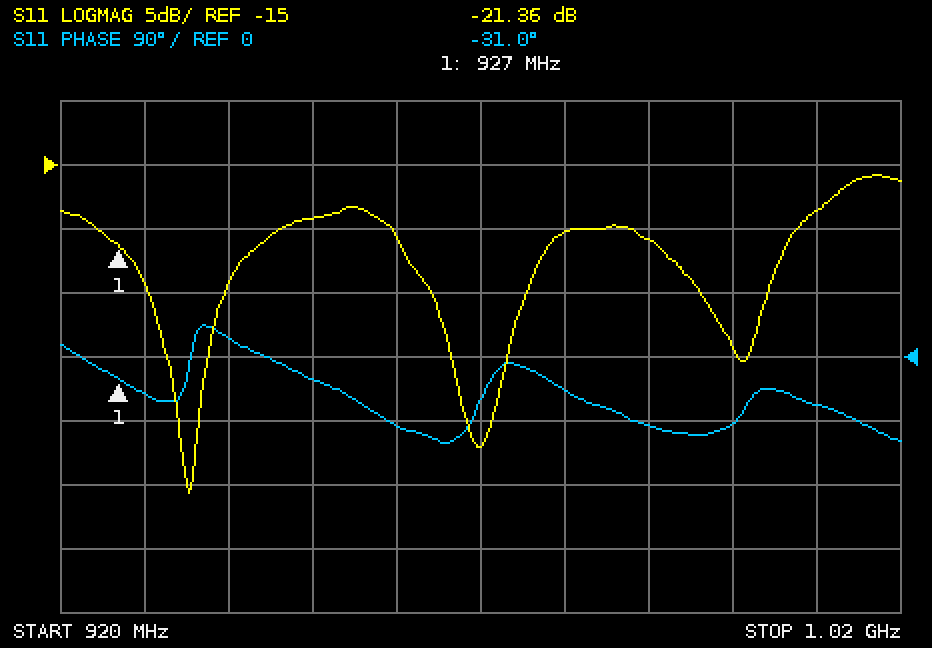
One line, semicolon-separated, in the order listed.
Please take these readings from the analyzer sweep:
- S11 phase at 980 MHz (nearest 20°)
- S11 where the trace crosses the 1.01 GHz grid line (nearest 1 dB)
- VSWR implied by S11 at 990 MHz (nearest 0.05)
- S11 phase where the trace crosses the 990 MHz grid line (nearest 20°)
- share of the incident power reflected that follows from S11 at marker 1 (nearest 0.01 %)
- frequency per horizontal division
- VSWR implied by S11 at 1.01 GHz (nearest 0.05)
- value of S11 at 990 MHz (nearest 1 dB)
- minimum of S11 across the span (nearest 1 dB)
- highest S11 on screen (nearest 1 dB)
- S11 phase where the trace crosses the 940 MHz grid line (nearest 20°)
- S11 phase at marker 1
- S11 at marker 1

-40°; -19 dB; 1.20; -100°; 0.73 %; 10 MHz; 1.25; -21 dB; -41 dB; -16 dB; 20°; -31.0°; -21.36 dB
